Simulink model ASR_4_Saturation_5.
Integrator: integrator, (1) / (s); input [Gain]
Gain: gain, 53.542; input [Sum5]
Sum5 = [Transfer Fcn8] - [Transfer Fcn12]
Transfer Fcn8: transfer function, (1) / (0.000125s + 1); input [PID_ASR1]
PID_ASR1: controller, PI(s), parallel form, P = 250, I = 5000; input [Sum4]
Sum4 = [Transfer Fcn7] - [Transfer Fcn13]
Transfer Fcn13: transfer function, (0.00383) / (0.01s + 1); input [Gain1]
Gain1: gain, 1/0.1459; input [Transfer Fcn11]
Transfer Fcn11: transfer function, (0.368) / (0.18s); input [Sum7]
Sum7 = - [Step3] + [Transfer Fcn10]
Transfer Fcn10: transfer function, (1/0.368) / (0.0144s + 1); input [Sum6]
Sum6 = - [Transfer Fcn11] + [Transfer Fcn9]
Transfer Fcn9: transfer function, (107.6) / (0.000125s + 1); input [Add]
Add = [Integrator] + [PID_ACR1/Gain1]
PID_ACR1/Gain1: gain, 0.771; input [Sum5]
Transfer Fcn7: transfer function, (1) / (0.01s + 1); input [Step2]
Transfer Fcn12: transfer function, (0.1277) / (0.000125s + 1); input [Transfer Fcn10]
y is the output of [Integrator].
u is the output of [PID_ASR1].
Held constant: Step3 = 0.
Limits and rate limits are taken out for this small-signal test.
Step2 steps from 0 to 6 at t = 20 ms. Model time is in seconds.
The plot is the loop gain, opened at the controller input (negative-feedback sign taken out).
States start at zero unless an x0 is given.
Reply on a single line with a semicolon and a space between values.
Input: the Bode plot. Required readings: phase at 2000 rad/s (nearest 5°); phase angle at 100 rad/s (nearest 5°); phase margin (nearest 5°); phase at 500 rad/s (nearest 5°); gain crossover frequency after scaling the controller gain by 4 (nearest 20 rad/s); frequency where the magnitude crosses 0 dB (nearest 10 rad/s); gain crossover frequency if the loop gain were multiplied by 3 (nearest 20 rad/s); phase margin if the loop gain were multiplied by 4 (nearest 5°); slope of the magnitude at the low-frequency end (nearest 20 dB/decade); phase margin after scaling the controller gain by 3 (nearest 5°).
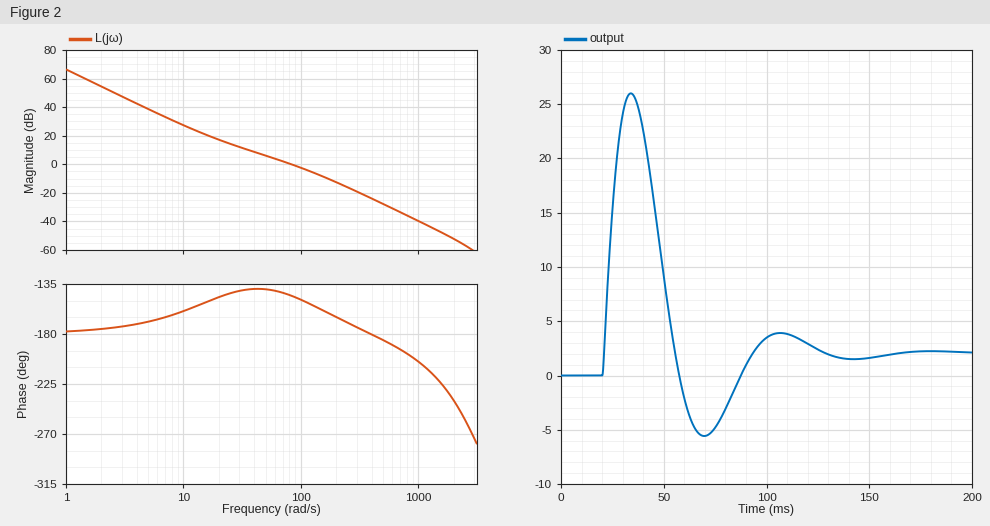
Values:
-240°; -150°; 35°; -185°; 200 rad/s; 80 rad/s; 160 rad/s; 15°; -40 dB/decade; 20°
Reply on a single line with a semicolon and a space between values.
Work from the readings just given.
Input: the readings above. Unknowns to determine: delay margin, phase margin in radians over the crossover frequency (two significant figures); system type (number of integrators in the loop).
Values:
0.0076 s; 2
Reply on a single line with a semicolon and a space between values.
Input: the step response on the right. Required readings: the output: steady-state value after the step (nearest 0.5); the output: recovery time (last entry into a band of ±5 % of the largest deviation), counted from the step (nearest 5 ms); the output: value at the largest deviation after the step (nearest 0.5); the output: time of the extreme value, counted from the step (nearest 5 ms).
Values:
2.0; 95 ms; 26.0; 15 ms
